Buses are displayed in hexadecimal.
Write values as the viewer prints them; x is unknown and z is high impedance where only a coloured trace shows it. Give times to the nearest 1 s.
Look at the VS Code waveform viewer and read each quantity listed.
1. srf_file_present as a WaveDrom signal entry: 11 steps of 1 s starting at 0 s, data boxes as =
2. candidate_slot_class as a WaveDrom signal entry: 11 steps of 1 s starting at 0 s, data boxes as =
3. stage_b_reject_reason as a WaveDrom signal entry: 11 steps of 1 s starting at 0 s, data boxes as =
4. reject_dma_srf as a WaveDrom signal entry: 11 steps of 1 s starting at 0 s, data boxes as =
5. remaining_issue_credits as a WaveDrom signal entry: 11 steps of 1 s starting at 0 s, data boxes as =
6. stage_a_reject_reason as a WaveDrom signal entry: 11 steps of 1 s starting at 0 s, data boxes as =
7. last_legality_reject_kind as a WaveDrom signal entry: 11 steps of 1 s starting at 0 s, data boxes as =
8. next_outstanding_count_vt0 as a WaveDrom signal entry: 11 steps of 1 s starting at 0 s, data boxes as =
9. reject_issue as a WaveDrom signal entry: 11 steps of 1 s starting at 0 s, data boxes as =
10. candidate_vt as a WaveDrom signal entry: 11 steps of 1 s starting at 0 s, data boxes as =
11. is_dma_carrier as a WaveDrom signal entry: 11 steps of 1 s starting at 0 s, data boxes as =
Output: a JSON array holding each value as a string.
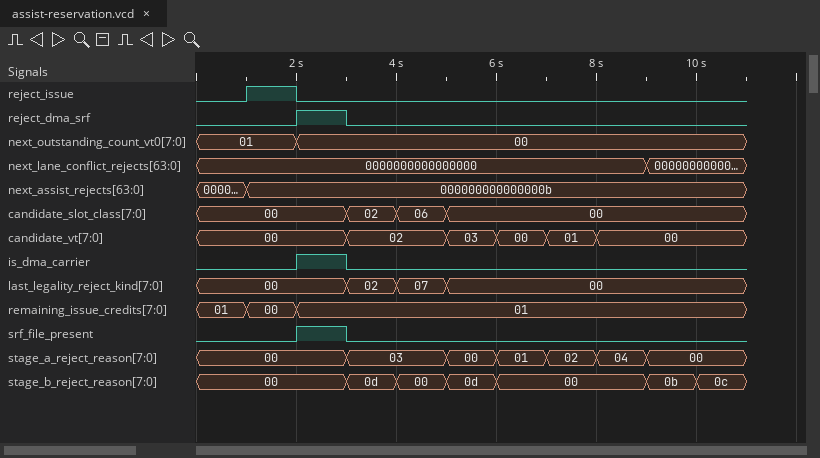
["{name: 'srf_file_present', wave: '0.10.......'}", "{name: 'candidate_slot_class', wave: '=..===.....', data: '00 02 06 00'}", "{name: 'stage_b_reject_reason', wave: '=..====..==', data: '00 0d 00 0d 00 0b 0c'}", "{name: 'reject_dma_srf', wave: '0.10.......'}", "{name: 'remaining_issue_credits', wave: '===........', data: '01 00 01'}", "{name: 'stage_a_reject_reason', wave: '=..=.=====.', data: '00 03 00 01 02 04 00'}", "{name: 'last_legality_reject_kind', wave: '=..===.....', data: '00 02 07 00'}", "{name: 'next_outstanding_count_vt0', wave: '=.=........', data: '01 00'}", "{name: 'reject_issue', wave: '010........'}", "{name: 'candidate_vt', wave: '=..=.====..', data: '00 02 03 00 01 00'}", "{name: 'is_dma_carrier', wave: '0.10.......'}"]
